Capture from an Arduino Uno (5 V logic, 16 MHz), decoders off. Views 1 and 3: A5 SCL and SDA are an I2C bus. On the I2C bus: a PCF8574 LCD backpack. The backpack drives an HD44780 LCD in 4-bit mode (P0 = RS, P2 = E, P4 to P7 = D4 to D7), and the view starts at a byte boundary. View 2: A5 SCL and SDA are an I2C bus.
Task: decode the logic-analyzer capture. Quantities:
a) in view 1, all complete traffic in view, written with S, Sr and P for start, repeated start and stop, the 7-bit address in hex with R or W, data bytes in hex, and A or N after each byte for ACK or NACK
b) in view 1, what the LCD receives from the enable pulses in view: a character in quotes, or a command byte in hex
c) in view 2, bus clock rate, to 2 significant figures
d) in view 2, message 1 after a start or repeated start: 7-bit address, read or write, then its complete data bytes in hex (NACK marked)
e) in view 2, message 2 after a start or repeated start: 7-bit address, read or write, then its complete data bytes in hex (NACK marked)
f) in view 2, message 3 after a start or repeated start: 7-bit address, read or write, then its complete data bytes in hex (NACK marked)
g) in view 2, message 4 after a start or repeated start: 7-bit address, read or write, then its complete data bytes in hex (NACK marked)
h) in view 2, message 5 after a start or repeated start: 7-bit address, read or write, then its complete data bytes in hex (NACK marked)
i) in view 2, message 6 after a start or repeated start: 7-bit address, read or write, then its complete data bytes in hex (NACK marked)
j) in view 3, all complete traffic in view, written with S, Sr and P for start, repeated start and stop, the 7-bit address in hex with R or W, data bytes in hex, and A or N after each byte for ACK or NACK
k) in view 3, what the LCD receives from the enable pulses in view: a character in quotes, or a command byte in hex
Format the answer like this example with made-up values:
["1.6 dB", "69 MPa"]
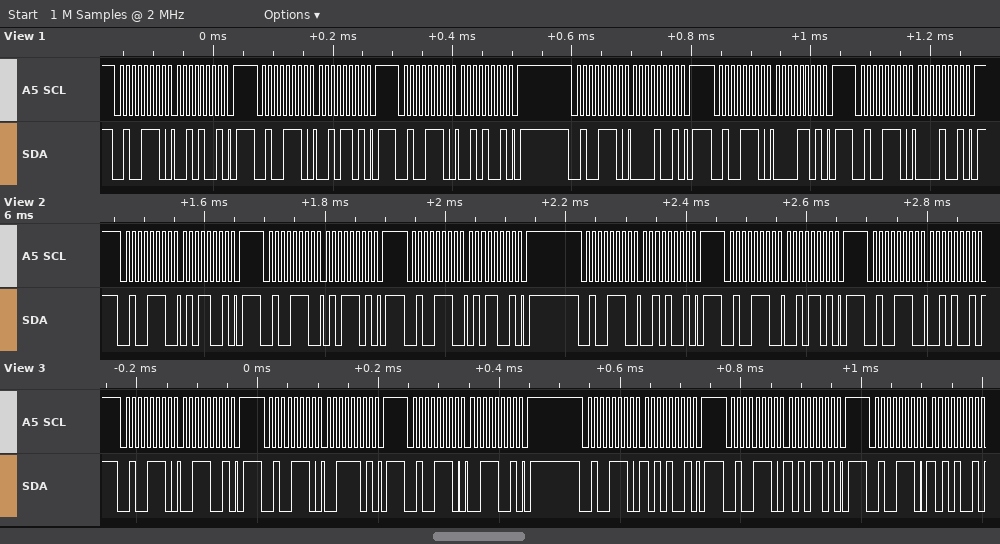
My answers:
["S 27W A 29 A P S 27W A 2D A P S 27W A 29 A P S 27W A 09 A P S 27W A 0D A P S 27W A 09 A P", "' '", "100 kHz", "0x27 write: 59", "0x27 write: 5D", "0x27 write: 59", "0x27 write: 29", "0x27 write: 2D", "0x27 write: 29", "S 27W A 39 A P S 27W A 3D A P S 27W A 39 A P S 27W A A9 A P S 27W A AD A P S 27W A A9 A", "':'"]
